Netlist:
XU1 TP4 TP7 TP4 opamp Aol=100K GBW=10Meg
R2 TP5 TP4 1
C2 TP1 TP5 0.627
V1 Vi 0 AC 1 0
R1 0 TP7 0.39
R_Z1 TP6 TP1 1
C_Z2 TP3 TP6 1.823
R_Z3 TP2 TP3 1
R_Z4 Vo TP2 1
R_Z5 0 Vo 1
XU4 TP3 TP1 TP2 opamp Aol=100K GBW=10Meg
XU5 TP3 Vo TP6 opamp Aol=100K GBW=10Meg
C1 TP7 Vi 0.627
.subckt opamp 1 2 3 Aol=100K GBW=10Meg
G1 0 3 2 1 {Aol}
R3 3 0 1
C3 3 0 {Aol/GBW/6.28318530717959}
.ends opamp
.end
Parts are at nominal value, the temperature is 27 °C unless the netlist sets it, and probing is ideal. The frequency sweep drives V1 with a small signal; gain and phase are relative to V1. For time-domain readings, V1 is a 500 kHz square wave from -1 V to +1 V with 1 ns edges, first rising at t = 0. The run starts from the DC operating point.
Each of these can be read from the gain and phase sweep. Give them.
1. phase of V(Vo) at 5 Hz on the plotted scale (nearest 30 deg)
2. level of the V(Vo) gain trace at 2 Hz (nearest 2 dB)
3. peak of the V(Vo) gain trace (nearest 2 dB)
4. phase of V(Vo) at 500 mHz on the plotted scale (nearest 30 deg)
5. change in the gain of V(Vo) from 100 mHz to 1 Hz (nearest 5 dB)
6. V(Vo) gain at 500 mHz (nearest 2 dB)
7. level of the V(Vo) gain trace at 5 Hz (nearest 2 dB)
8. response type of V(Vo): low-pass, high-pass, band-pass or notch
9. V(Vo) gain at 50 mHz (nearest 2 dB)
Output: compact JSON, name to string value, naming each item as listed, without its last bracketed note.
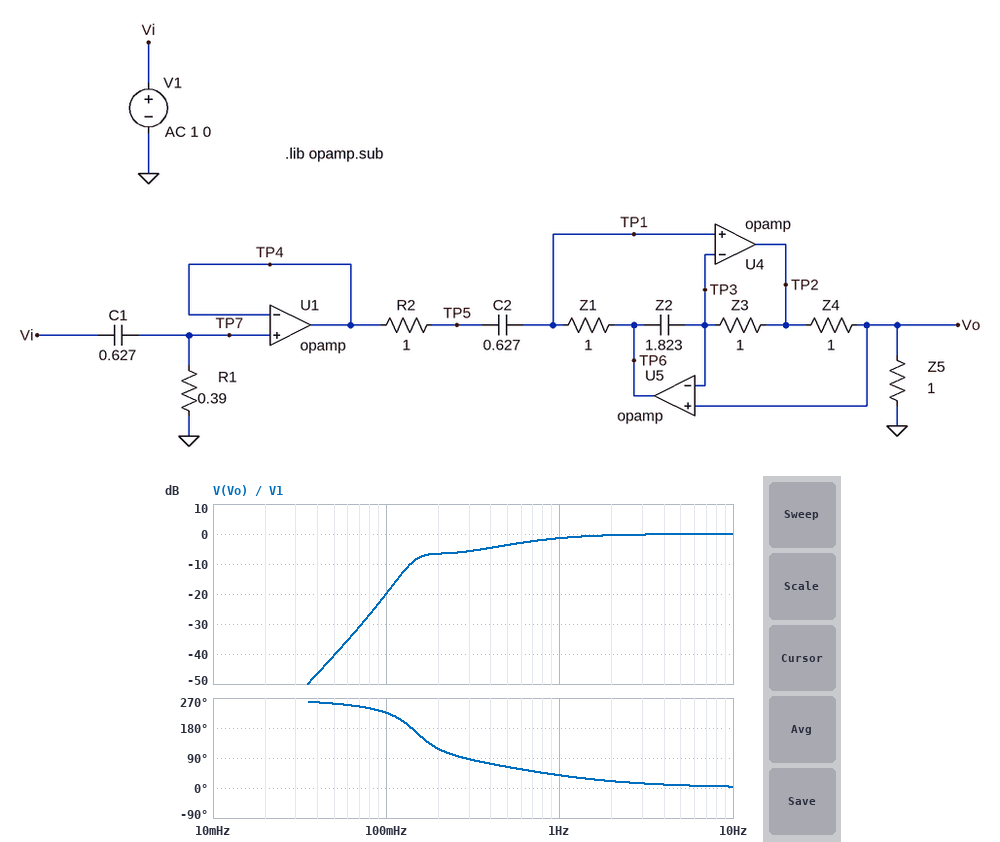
{"phase of V(Vo) at 5 Hz on the plotted scale": "0 deg", "level of the V(Vo) gain trace at 2 Hz": "0 dB", "peak of the V(Vo) gain trace": "0 dB", "phase of V(Vo) at 500 mHz on the plotted scale": "60 deg", "change in the gain of V(Vo) from 100 mHz to 1 Hz": "20 dB", "V(Vo) gain at 500 mHz": "-4 dB", "level of the V(Vo) gain trace at 5 Hz": "0 dB", "response type of V(Vo): low-pass, high-pass, band-pass or notch": "high-pass", "V(Vo) gain at 50 mHz": "-40 dB"}
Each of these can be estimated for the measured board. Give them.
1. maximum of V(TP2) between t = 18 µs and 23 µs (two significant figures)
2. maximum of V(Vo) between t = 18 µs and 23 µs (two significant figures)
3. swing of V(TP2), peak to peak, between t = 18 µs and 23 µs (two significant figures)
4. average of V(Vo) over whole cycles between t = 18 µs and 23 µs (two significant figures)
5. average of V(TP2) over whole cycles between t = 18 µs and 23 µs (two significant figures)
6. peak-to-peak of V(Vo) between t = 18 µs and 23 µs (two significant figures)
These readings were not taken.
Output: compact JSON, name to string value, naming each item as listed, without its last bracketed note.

{"maximum of V(TP2) between t = 18 µs and 23 µs": "4.0 V", "maximum of V(Vo) between t = 18 µs and 23 µs": "2.0 V", "swing of V(TP2), peak to peak, between t = 18 µs and 23 µs": "4.0 V", "average of V(Vo) over whole cycles between t = 18 µs and 23 µs": "1.0 V", "average of V(TP2) over whole cycles between t = 18 µs and 23 µs": "2.0 V", "peak-to-peak of V(Vo) between t = 18 µs and 23 µs": "2.0 V"}
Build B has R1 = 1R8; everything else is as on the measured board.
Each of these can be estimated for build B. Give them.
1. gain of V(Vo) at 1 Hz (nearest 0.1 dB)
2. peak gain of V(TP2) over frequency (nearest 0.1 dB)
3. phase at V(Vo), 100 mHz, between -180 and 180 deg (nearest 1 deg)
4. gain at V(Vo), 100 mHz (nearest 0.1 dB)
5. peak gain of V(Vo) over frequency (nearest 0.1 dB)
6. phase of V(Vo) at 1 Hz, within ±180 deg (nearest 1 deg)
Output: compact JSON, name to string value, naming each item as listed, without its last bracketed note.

{"gain of V(Vo) at 1 Hz": "0.1 dB", "peak gain of V(TP2) over frequency": "8.7 dB", "phase at V(Vo), 100 mHz, between -180 and 180 deg": "-161 deg", "gain at V(Vo), 100 mHz": "-8.3 dB", "peak gain of V(Vo) over frequency": "2.7 dB", "phase of V(Vo) at 1 Hz, within ±180 deg": "13 deg"}
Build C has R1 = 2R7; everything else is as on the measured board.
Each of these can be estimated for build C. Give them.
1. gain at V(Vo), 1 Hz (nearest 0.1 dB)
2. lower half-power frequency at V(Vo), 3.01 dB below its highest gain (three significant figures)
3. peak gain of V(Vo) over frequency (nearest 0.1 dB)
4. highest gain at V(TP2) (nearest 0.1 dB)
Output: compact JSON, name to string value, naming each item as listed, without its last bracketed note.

{"gain at V(Vo), 1 Hz": "0.1 dB", "lower half-power frequency at V(Vo), 3.01 dB below its highest gain": "130 mHz", "peak gain of V(Vo) over frequency": "3.8 dB", "highest gain at V(TP2)": "9.8 dB"}
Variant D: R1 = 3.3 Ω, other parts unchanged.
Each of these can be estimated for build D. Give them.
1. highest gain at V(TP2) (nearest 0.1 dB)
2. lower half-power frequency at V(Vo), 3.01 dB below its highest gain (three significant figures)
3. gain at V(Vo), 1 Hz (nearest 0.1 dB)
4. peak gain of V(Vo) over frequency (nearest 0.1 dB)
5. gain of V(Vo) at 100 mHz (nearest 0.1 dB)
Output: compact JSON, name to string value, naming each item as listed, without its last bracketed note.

{"highest gain at V(TP2)": "10.2 dB", "lower half-power frequency at V(Vo), 3.01 dB below its highest gain": "129 mHz", "gain at V(Vo), 1 Hz": "0.1 dB", "peak gain of V(Vo) over frequency": "4.2 dB", "gain of V(Vo) at 100 mHz": "-5.5 dB"}
